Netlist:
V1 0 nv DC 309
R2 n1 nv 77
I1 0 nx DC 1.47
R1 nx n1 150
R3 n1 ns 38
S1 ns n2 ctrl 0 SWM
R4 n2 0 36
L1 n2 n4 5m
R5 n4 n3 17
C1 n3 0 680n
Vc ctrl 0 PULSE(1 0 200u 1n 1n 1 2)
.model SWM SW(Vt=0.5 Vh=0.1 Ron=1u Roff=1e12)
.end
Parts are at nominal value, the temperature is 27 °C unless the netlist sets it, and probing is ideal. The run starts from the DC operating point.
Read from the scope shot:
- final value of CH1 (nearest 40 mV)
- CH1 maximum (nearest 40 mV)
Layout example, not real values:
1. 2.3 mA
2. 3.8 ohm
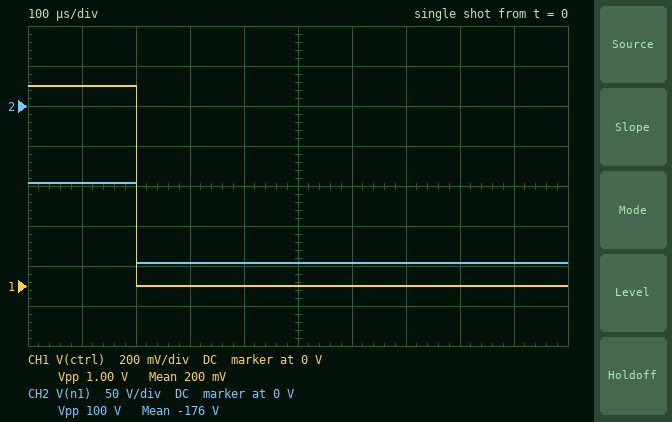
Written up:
1. 0 V
2. 1.00 V
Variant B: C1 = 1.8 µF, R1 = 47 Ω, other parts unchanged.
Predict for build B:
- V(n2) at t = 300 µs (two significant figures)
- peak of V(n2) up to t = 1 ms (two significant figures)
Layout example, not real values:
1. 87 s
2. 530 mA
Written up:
1. -17 V
2. 2.8 V
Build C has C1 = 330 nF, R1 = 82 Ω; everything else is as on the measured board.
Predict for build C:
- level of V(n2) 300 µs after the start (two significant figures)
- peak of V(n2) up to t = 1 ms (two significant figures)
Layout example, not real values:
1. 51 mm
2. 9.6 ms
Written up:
1. -5.5 V
2. 5.1 V
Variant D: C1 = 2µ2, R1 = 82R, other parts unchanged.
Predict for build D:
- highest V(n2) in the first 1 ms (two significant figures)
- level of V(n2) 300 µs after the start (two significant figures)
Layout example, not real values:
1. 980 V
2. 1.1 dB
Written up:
1. 2.2 V
2. -18 V
